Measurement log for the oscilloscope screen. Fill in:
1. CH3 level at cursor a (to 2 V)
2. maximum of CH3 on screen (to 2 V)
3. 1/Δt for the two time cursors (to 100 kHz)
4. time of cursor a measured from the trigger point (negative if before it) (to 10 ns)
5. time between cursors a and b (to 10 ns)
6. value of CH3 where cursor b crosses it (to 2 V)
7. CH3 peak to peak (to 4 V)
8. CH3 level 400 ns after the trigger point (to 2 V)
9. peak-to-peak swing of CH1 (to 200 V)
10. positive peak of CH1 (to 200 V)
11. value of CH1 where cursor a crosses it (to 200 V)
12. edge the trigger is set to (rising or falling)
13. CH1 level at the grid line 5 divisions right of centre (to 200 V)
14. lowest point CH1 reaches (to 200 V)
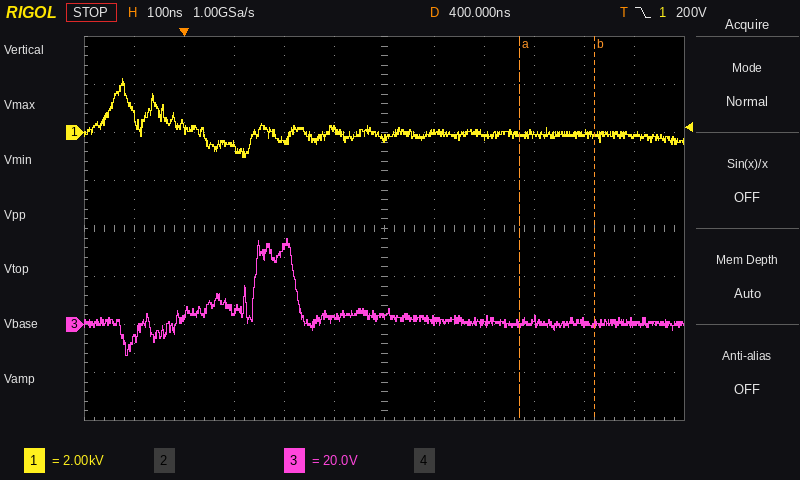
0 V
36 V
6.7 MHz
+670 ns
150 ns
0 V
48 V
4 V
3.2 kV
2.2 kV
0.0 kV
falling
-200 V
-1.0 kV
